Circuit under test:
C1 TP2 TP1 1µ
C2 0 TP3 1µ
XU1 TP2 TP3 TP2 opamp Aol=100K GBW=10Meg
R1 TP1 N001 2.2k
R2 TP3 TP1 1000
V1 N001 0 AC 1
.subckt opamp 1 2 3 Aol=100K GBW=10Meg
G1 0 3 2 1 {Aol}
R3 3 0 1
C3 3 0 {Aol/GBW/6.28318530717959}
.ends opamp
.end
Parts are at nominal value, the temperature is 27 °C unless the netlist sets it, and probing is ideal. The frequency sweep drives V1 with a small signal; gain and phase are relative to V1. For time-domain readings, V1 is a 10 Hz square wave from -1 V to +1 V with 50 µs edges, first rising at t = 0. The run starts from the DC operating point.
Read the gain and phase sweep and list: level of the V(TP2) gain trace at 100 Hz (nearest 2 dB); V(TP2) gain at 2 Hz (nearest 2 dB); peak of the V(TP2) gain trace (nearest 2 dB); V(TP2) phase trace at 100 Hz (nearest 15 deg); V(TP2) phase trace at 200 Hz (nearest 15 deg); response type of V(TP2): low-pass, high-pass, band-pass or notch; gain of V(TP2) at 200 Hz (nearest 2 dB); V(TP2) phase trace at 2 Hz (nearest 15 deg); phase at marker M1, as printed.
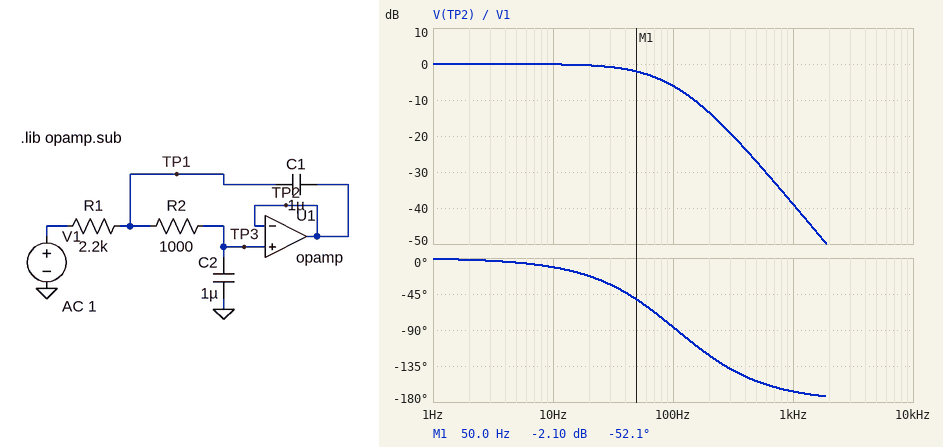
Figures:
-6 dB
0 dB
0 dB
-90 deg
-120 deg
low-pass
-14 dB
0 deg
-52.1 deg
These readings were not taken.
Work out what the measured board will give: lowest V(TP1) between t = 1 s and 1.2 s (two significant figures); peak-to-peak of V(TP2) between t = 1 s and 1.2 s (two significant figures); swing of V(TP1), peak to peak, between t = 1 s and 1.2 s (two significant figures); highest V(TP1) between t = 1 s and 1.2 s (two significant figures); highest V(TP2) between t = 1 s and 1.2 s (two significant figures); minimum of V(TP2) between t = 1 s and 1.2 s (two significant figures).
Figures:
-1.0 V
2.0 V
2.0 V
1.0 V
1.0 V
-1.0 V
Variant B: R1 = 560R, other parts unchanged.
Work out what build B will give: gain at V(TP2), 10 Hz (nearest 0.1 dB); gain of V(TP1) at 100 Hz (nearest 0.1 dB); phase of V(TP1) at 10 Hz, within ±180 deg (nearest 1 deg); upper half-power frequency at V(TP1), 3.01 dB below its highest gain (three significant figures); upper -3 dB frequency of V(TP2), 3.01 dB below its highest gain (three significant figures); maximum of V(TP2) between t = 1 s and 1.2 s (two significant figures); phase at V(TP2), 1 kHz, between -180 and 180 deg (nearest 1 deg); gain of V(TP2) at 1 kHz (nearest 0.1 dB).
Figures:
0 dB
-0.5 dB
-2 deg
284 Hz
129 Hz
1.0 V
-155 deg
-27.3 dB
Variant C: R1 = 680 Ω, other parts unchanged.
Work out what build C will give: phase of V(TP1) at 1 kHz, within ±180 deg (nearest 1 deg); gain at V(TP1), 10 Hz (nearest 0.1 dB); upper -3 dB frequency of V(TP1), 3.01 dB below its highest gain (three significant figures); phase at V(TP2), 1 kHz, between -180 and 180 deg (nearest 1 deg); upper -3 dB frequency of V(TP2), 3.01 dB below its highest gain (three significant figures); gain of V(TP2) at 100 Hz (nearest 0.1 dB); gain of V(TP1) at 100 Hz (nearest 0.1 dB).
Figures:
-77 deg
0 dB
234 Hz
-158 deg
121 Hz
-2.2 dB
-0.7 dB
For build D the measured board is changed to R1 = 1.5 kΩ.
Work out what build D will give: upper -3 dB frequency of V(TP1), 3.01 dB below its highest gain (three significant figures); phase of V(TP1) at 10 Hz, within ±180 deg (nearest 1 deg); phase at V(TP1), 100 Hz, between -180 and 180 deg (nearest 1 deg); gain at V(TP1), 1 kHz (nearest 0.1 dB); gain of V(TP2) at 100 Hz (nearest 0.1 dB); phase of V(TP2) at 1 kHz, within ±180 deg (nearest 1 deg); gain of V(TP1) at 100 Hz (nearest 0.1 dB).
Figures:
106 Hz
-5 deg
-43 deg
-19.5 dB
-4.2 dB
-165 deg
-2.8 dB
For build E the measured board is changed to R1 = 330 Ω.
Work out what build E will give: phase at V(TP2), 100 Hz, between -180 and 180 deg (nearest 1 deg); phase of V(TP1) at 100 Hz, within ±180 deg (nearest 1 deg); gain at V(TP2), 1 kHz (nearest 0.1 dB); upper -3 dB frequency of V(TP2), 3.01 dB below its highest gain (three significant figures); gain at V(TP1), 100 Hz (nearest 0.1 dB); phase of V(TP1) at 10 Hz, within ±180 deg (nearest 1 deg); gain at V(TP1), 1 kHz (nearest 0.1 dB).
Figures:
-44 deg
-12 deg
-23.3 dB
145 Hz
-0.2 dB
-1 deg
-7.2 dB
